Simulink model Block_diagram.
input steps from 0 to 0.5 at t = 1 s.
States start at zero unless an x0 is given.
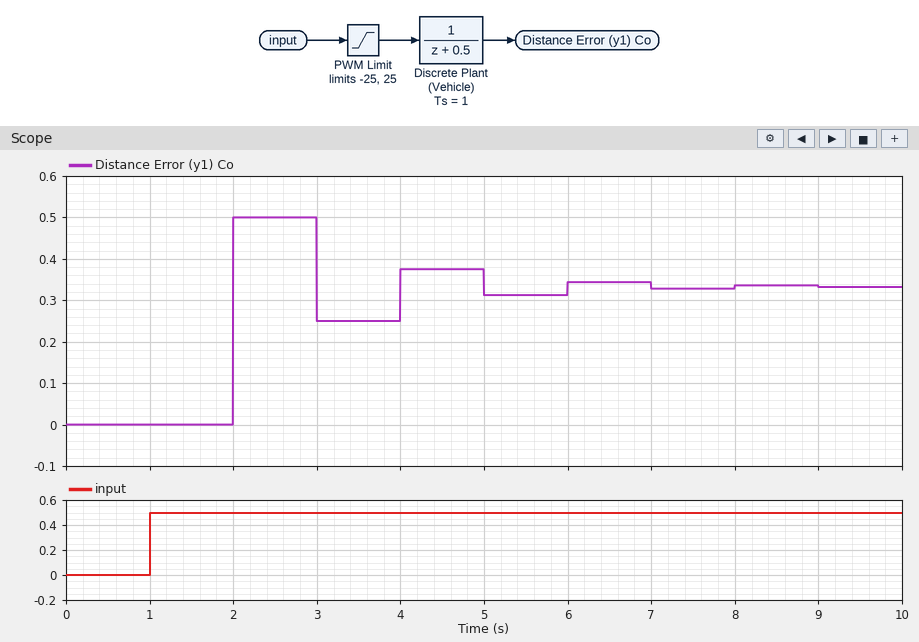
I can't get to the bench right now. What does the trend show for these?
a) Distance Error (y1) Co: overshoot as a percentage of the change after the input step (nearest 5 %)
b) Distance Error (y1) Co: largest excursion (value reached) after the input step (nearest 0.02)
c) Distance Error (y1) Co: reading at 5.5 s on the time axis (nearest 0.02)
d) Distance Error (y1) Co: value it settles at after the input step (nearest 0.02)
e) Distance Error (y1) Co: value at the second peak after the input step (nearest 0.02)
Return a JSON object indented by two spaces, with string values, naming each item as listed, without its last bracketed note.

{
  "Distance Error (y1) Co: overshoot as a percentage of the change after the input step": "50 %",
  "Distance Error (y1) Co: largest excursion (value reached) after the input step": "0.50",
  "Distance Error (y1) Co: reading at 5.5 s on the time axis": "0.32",
  "Distance Error (y1) Co: value it settles at after the input step": "0.34",
  "Distance Error (y1) Co: value at the second peak after the input step": "0.38"
}
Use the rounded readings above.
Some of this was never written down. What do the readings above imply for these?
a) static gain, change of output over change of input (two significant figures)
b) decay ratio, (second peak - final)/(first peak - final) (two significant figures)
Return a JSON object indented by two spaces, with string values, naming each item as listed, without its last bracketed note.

{
  "static gain, change of output over change of input": "0.68",
  "decay ratio, (second peak - final)/(first peak - final)": "0.25"
}
